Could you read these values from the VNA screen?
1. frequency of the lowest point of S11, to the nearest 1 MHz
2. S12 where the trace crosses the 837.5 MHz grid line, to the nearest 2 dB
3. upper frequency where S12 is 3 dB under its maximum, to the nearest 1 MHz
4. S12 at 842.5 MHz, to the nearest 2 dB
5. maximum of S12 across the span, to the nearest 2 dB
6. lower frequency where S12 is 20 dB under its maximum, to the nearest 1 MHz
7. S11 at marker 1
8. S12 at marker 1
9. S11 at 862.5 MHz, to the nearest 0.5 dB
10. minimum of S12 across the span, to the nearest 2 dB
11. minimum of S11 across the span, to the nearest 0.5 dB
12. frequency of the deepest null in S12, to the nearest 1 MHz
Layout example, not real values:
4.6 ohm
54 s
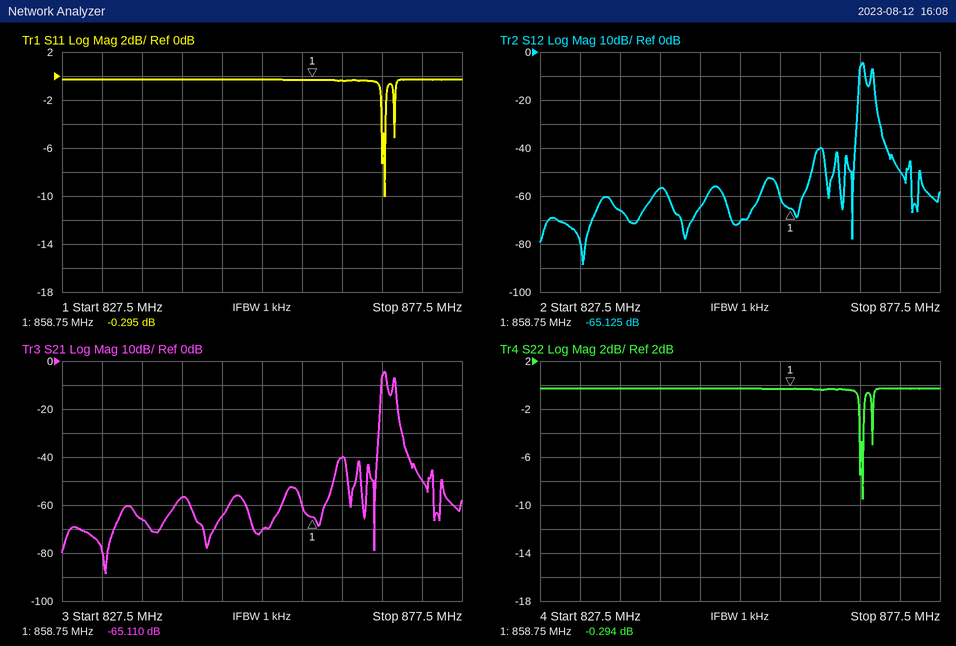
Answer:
868 MHz
-66 dB
868 MHz
-56 dB
-4 dB
867 MHz
-0.295 dB
-65.125 dB
-0.5 dB
-88 dB
-10.0 dB
833 MHz
